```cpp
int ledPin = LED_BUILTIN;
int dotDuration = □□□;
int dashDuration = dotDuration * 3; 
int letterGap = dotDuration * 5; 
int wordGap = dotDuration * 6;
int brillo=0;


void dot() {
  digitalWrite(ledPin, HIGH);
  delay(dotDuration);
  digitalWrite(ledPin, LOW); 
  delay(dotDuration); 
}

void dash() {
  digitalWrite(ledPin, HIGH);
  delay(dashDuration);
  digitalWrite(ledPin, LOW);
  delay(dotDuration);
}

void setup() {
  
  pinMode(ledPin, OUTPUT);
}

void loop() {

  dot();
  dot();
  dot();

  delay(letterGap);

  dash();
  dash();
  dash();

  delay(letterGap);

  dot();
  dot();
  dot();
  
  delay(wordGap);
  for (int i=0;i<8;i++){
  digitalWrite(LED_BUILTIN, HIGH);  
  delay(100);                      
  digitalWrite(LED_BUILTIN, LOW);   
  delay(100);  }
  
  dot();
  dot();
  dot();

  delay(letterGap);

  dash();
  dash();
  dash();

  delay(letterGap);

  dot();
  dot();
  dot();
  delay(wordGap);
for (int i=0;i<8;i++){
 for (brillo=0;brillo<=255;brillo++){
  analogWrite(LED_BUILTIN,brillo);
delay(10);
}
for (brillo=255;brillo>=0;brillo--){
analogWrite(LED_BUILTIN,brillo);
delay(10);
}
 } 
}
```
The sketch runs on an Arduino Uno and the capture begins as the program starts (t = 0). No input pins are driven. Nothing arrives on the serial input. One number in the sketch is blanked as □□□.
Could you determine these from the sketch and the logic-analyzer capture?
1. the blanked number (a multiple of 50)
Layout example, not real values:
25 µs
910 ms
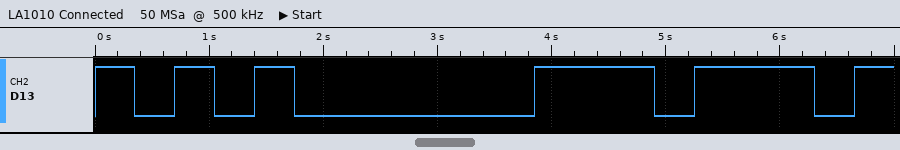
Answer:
350
